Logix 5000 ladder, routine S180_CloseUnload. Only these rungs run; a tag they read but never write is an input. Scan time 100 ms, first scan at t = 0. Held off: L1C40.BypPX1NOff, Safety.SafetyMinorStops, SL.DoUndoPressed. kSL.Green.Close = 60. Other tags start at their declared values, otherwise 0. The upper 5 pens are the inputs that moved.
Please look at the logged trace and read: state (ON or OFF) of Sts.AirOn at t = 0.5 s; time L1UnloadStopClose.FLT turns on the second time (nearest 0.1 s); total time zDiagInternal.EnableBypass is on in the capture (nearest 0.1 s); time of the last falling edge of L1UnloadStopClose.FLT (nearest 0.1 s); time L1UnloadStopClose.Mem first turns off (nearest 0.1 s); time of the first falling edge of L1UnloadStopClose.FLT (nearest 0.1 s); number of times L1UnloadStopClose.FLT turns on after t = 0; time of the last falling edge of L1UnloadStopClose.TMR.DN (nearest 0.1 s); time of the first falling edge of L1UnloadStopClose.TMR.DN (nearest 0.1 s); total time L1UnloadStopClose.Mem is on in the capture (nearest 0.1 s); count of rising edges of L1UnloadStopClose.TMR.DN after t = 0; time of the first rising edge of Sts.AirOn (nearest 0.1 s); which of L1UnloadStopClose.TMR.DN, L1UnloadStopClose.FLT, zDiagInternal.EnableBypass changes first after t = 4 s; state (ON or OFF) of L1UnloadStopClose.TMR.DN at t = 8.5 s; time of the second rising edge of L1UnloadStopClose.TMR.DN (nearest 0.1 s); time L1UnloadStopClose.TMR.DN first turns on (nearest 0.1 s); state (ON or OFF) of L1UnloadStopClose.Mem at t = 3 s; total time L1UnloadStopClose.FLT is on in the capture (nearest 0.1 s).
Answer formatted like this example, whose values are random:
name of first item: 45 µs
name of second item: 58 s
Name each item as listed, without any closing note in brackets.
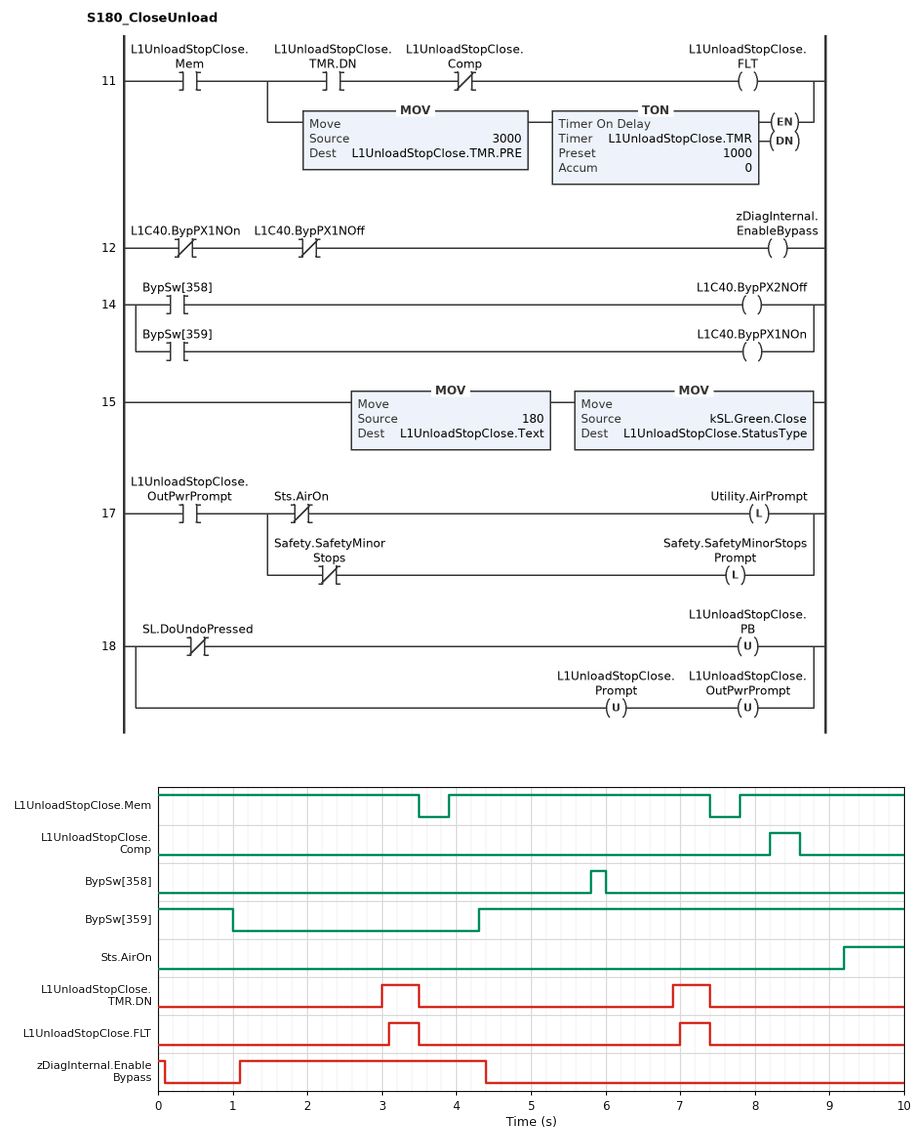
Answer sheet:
state (ON or OFF) of Sts.AirOn at t = 0.5 s: OFF
time L1UnloadStopClose.FLT turns on the second time: 7.0 s
total time zDiagInternal.EnableBypass is on in the capture: 3.4 s
time of the last falling edge of L1UnloadStopClose.FLT: 7.4 s
time L1UnloadStopClose.Mem first turns off: 3.5 s
time of the first falling edge of L1UnloadStopClose.FLT: 3.5 s
number of times L1UnloadStopClose.FLT turns on after t = 0: 2
time of the last falling edge of L1UnloadStopClose.TMR.DN: 7.4 s
time of the first falling edge of L1UnloadStopClose.TMR.DN: 3.5 s
total time L1UnloadStopClose.Mem is on in the capture: 9.2 s
count of rising edges of L1UnloadStopClose.TMR.DN after t = 0: 2
time of the first rising edge of Sts.AirOn: 9.2 s
which of L1UnloadStopClose.TMR.DN, L1UnloadStopClose.FLT, zDiagInternal.EnableBypass changes first after t = 4 s: zDiagInternal.EnableBypass
state (ON or OFF) of L1UnloadStopClose.TMR.DN at t = 8.5 s: OFF
time of the second rising edge of L1UnloadStopClose.TMR.DN: 6.9 s
time L1UnloadStopClose.TMR.DN first turns on: 3.0 s
state (ON or OFF) of L1UnloadStopClose.Mem at t = 3 s: ON
total time L1UnloadStopClose.FLT is on in the capture: 0.8 s
